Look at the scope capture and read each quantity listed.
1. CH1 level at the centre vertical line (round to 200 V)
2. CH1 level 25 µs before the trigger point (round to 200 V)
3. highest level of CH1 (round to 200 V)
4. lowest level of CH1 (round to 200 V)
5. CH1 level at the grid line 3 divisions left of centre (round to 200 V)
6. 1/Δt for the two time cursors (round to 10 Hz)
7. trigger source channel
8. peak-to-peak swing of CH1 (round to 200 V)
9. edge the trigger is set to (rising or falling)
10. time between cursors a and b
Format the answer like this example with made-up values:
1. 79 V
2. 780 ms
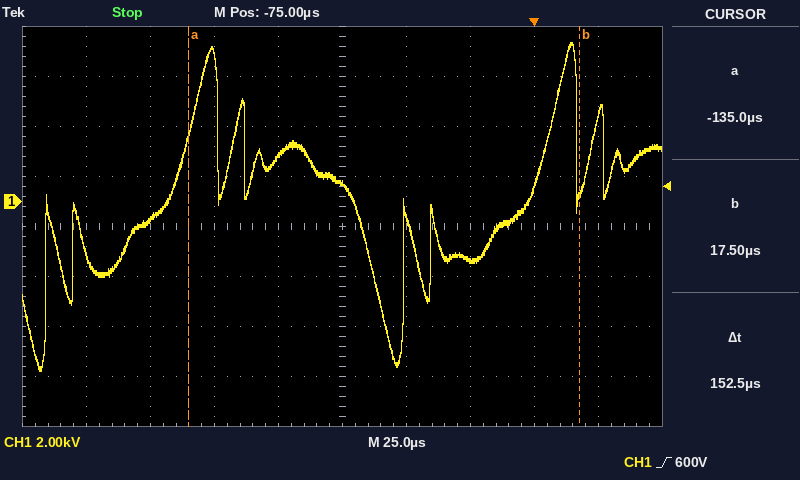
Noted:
1. 800 V
2. -2.4 kV
3. 6.4 kV
4. -6.8 kV
5. -800 V
6. 6.56 kHz
7. CH1
8. 13.2 kV
9. rising
10. 152.5 µs
